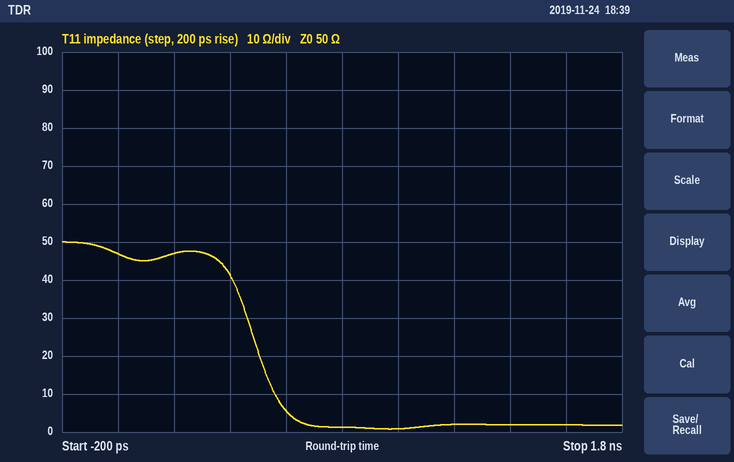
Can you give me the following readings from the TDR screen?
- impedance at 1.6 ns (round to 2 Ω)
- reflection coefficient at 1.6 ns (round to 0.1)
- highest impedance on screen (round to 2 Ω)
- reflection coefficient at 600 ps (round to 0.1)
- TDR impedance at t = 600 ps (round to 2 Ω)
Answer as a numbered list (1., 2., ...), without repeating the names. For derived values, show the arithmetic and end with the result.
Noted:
1. 2 Ω
2. (2 − 50)/(2 + 50) ≈ -0.9
3. 50 Ω
4. (6 − 50)/(6 + 50) ≈ -0.8
5. 6 Ω
